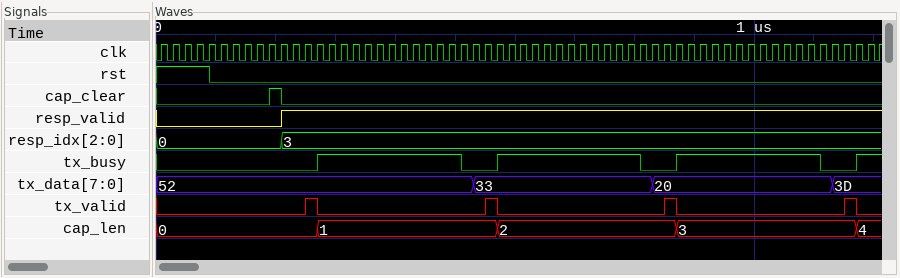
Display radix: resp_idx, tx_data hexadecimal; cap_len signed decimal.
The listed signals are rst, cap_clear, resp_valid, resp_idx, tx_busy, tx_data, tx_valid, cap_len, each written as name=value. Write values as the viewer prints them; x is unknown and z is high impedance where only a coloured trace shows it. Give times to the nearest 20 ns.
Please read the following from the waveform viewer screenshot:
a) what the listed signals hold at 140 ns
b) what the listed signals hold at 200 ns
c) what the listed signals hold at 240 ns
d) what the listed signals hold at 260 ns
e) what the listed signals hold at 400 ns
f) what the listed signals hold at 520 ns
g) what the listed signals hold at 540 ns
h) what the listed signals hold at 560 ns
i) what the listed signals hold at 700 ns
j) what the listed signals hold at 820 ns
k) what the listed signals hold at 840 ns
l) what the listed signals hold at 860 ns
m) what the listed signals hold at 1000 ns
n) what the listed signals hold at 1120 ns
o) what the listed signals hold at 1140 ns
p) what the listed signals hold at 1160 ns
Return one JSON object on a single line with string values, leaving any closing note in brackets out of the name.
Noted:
{"what the listed signals hold at 140 ns": "rst=0, cap_clear=0, resp_valid=0, resp_idx=0, tx_busy=0, tx_data=52, tx_valid=0, cap_len=0", "what the listed signals hold at 200 ns": "rst=0, cap_clear=1, resp_valid=0, resp_idx=0, tx_busy=0, tx_data=52, tx_valid=0, cap_len=0", "what the listed signals hold at 240 ns": "rst=0, cap_clear=0, resp_valid=1, resp_idx=3, tx_busy=0, tx_data=52, tx_valid=0, cap_len=0", "what the listed signals hold at 260 ns": "rst=0, cap_clear=0, resp_valid=1, resp_idx=3, tx_busy=0, tx_data=52, tx_valid=1, cap_len=0", "what the listed signals hold at 400 ns": "rst=0, cap_clear=0, resp_valid=1, resp_idx=3, tx_busy=1, tx_data=52, tx_valid=0, cap_len=1", "what the listed signals hold at 520 ns": "rst=0, cap_clear=0, resp_valid=1, resp_idx=3, tx_busy=0, tx_data=52, tx_valid=0, cap_len=1", "what the listed signals hold at 540 ns": "rst=0, cap_clear=0, resp_valid=1, resp_idx=3, tx_busy=0, tx_data=33, tx_valid=0, cap_len=1", "what the listed signals hold at 560 ns": "rst=0, cap_clear=0, resp_valid=1, resp_idx=3, tx_busy=0, tx_data=33, tx_valid=1, cap_len=1", "what the listed signals hold at 700 ns": "rst=0, cap_clear=0, resp_valid=1, resp_idx=3, tx_busy=1, tx_data=33, tx_valid=0, cap_len=2", "what the listed signals hold at 820 ns": "rst=0, cap_clear=0, resp_valid=1, resp_idx=3, tx_busy=0, tx_data=33, tx_valid=0, cap_len=2", "what the listed signals hold at 840 ns": "rst=0, cap_clear=0, resp_valid=1, resp_idx=3, tx_busy=0, tx_data=20, tx_valid=0, cap_len=2", "what the listed signals hold at 860 ns": "rst=0, cap_clear=0, resp_valid=1, resp_idx=3, tx_busy=0, tx_data=20, tx_valid=1, cap_len=2", "what the listed signals hold at 1000 ns": "rst=0, cap_clear=0, resp_valid=1, resp_idx=3, tx_busy=1, tx_data=20, tx_valid=0, cap_len=3", "what the listed signals hold at 1120 ns": "rst=0, cap_clear=0, resp_valid=1, resp_idx=3, tx_busy=0, tx_data=20, tx_valid=0, cap_len=3", "what the listed signals hold at 1140 ns": "rst=0, cap_clear=0, resp_valid=1, resp_idx=3, tx_busy=0, tx_data=3D, tx_valid=0, cap_len=3", "what the listed signals hold at 1160 ns": "rst=0, cap_clear=0, resp_valid=1, resp_idx=3, tx_busy=0, tx_data=3D, tx_valid=1, cap_len=3"}
